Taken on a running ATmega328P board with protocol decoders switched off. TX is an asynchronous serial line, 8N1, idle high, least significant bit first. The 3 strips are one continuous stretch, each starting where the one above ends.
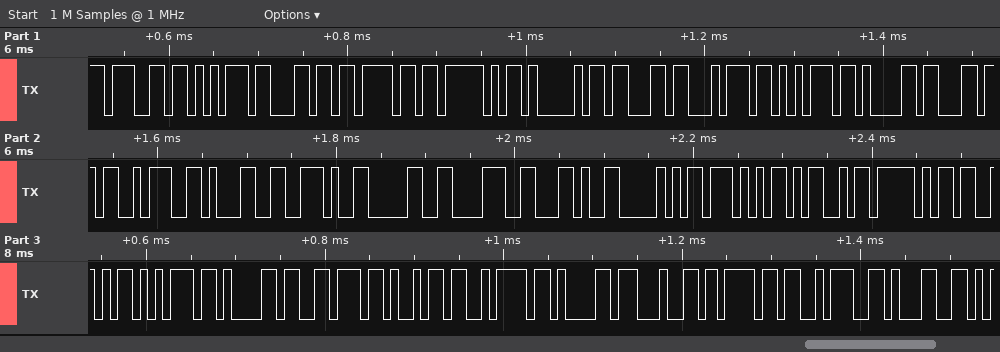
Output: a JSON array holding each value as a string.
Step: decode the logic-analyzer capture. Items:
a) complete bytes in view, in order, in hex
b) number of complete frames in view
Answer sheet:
["67 75 6C 6F 5F 41 63 74 75 61 6C 3A 31 2E 30 38 2C 50 57 4D 5F 53 75 61 76 69 7A 61 64 6F 3A 31", "32"]
